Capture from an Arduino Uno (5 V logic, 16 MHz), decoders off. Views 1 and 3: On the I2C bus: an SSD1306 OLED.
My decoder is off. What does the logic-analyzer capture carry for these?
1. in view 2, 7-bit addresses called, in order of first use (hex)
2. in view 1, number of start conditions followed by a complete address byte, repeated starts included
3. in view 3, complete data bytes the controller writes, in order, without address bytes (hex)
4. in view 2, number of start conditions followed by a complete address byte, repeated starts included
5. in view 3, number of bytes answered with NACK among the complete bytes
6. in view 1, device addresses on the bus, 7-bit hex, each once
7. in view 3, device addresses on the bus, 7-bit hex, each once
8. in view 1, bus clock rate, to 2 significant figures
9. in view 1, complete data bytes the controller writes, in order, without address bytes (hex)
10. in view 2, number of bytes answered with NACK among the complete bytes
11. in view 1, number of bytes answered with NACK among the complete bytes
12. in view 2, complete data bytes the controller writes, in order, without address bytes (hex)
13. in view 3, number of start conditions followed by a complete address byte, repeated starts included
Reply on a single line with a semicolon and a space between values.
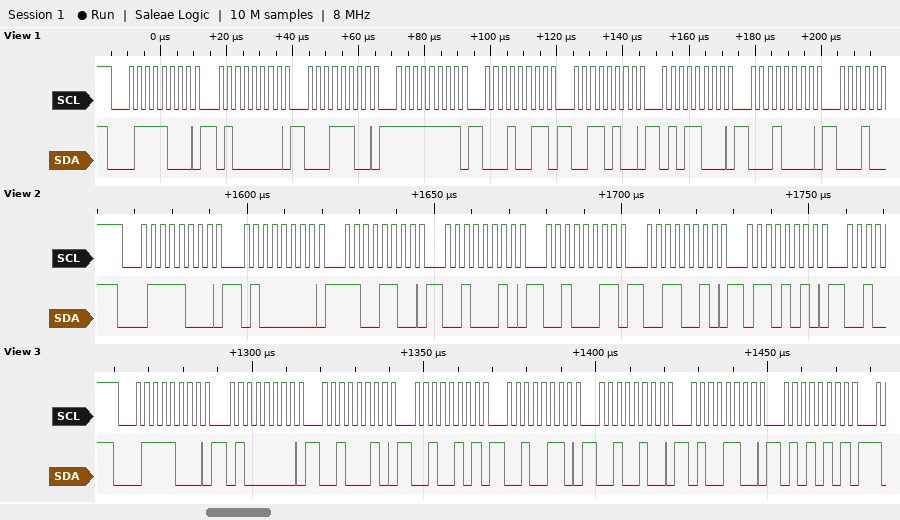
0x3C; 1; 40 22 25 26 24 4C 55; 1; 0; 0x3C; 0x3C; 400 kHz; 40 1C FF 13 34 58 10; 0; 0; 40 CC 22 23 32 6A; 1
